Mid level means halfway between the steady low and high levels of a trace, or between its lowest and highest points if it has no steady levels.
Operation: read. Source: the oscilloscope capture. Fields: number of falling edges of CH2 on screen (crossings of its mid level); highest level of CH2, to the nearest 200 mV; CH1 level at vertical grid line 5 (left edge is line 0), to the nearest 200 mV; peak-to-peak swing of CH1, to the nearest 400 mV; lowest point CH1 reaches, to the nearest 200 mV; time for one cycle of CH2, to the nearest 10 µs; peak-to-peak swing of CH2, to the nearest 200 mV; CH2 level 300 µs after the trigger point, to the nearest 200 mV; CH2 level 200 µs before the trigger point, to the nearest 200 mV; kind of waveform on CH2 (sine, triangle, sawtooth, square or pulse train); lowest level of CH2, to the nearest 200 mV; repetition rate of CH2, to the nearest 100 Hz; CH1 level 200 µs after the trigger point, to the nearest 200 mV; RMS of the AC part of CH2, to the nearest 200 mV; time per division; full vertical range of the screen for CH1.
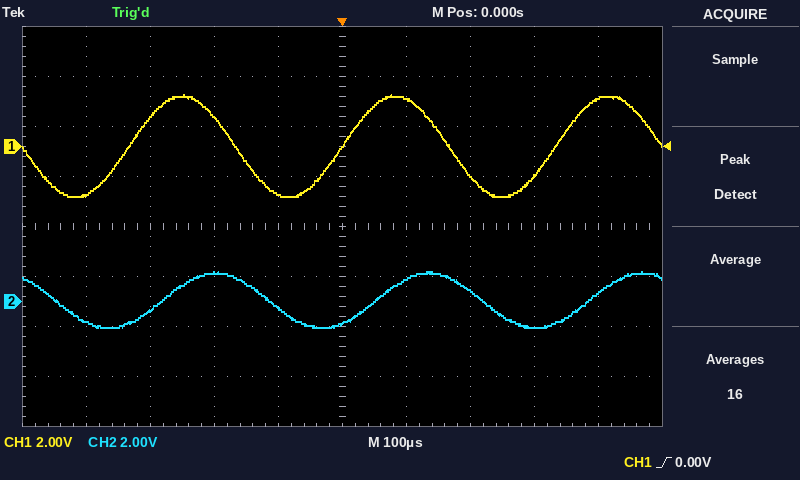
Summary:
3
1.2 V
0.0 V
4.0 V
-2.0 V
330 µs
2.2 V
-1.0 V
1.2 V
sine
-1.0 V
3.0 kHz
-1.2 V
800 mV
100 µs
16 V
